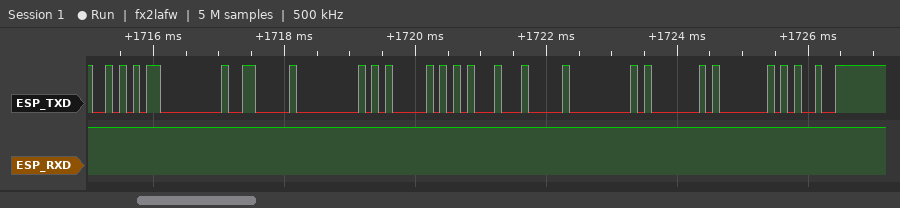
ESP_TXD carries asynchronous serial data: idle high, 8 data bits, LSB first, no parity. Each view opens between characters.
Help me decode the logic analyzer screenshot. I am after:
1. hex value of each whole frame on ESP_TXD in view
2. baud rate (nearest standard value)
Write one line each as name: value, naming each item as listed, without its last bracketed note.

hex value of each whole frame on ESP_TXD in view: AA, 00, 06, 00, 05, 15, 04, 00, 01, 01, 25
baud rate: 9600 baud
